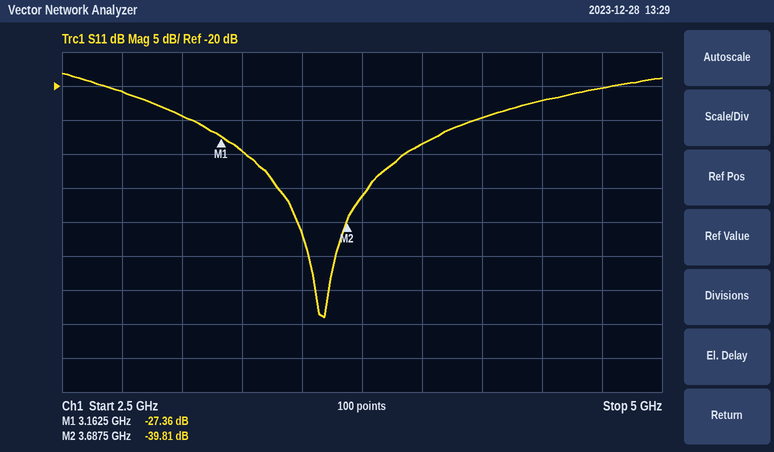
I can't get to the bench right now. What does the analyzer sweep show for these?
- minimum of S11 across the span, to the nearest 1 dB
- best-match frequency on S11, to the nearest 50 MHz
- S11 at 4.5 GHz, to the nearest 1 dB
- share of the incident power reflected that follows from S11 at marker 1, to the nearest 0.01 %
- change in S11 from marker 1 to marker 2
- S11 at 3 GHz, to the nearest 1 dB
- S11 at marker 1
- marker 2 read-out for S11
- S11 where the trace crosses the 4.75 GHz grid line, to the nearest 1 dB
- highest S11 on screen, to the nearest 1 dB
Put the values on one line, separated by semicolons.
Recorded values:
-54 dB; 3.60 GHz; -22 dB; 0.18 %; -12.45 dB; -24 dB; -27.36 dB; -39.81 dB; -20 dB; -18 dB
